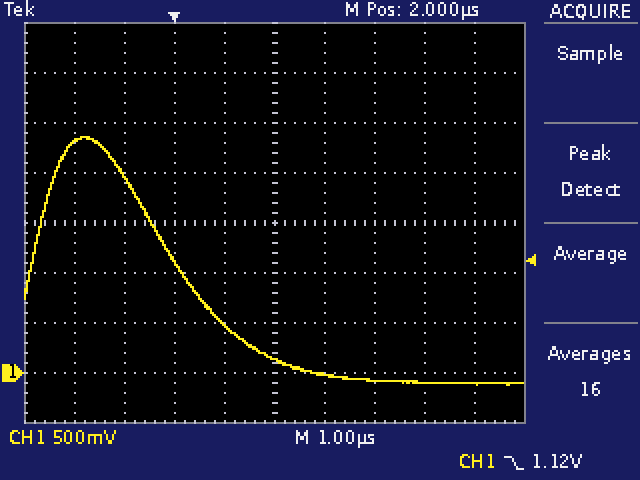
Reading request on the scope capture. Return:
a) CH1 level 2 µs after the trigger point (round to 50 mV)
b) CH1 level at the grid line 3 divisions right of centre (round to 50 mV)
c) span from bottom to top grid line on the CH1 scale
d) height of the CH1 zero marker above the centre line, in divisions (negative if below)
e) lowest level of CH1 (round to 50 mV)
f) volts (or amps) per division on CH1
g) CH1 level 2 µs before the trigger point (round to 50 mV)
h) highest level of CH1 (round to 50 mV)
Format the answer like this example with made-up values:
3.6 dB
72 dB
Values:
150 mV
-100 mV
4 V
-3.0 div
-100 mV
500 mV
2.30 V
2.35 V
